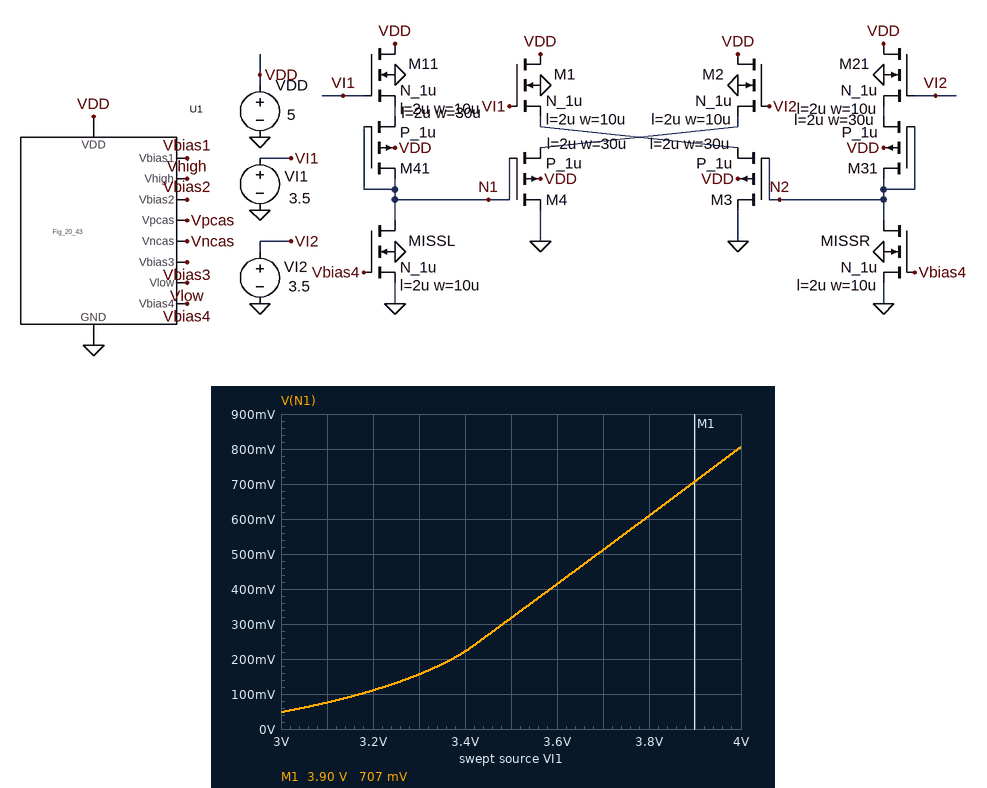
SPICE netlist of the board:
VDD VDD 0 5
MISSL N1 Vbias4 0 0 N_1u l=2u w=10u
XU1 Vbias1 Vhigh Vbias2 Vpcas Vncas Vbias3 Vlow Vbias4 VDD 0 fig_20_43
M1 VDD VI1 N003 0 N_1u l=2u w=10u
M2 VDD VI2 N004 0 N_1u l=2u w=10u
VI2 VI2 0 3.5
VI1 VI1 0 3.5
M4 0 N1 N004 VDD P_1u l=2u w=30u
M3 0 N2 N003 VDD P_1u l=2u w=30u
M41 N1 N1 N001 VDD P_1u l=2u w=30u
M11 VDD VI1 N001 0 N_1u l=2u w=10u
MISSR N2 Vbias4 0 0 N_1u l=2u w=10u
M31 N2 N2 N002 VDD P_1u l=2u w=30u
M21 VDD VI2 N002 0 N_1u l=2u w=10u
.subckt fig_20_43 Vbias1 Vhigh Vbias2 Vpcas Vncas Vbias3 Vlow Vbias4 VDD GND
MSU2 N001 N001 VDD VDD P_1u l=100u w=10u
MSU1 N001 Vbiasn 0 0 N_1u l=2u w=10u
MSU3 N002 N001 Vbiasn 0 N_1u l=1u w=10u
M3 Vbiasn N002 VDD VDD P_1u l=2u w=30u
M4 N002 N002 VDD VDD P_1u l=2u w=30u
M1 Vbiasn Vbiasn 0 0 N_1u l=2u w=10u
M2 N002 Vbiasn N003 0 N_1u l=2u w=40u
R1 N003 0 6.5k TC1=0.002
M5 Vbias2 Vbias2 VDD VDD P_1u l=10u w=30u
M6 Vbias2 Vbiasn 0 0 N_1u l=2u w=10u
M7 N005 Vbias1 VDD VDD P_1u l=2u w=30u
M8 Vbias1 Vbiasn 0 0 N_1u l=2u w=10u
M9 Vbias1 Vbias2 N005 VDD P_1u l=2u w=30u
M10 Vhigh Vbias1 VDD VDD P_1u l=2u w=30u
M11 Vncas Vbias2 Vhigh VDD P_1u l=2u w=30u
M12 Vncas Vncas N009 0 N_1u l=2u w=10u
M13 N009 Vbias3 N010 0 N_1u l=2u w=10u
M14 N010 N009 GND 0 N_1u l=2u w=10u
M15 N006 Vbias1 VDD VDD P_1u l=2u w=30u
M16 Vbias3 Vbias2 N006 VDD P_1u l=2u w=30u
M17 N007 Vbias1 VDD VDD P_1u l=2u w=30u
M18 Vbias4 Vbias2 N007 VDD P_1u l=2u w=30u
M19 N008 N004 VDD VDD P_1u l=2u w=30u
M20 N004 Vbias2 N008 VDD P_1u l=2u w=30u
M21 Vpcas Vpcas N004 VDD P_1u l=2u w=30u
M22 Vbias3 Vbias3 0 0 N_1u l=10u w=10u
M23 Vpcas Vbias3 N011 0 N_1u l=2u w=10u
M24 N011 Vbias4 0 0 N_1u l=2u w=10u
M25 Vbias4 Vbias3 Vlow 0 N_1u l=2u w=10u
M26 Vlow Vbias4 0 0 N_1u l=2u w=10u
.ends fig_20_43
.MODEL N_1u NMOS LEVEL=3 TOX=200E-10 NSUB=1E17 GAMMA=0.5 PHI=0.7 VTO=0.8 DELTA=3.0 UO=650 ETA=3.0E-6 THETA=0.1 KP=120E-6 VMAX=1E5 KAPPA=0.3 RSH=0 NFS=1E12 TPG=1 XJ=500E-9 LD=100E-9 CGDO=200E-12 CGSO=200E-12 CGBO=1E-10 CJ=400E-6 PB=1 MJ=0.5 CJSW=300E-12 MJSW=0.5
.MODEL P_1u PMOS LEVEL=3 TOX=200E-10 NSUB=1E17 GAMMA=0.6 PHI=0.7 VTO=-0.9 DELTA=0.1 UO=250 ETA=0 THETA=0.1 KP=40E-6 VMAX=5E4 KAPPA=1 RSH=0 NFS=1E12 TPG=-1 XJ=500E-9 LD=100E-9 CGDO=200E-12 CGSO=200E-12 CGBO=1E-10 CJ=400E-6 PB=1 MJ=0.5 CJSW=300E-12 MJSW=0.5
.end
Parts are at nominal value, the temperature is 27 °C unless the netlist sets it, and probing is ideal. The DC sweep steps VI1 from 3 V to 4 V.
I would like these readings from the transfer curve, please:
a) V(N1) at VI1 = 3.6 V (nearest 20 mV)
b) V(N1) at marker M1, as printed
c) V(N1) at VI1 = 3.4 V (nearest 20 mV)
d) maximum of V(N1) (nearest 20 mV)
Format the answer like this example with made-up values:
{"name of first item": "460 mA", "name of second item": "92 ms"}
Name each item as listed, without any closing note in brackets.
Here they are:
{"V(N1) at VI1 = 3.6 V": "420 mV", "V(N1) at marker M1, as printed": "707 mV", "V(N1) at VI1 = 3.4 V": "220 mV", "maximum of V(N1)": "800 mV"}
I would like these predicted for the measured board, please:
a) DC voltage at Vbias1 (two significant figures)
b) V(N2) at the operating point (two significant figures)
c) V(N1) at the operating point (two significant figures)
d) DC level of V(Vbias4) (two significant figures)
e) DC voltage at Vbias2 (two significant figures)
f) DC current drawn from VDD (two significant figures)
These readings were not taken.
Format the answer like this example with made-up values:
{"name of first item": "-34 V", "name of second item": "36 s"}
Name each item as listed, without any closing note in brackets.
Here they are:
{"DC voltage at Vbias1": "3.8 V", "V(N2) at the operating point": "320 mV", "V(N1) at the operating point": "320 mV", "DC level of V(Vbias4)": "1.1 V", "DC voltage at Vbias2": "3.4 V", "DC current drawn from VDD": "280 µA"}
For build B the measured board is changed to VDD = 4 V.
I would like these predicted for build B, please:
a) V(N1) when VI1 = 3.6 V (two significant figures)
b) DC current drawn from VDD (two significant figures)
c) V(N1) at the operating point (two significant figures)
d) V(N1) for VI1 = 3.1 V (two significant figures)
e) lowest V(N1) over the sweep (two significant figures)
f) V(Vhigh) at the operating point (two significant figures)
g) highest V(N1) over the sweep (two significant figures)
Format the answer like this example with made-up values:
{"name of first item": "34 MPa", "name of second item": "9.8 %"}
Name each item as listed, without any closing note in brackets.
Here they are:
{"V(N1) when VI1 = 3.6 V": "570 mV", "DC current drawn from VDD": "260 µA", "V(N1) at the operating point": "470 mV", "V(N1) for VI1 = 3.1 V": "130 mV", "lowest V(N1) over the sweep": "89 mV", "V(Vhigh) at the operating point": "3.7 V", "highest V(N1) over the sweep": "970 mV"}
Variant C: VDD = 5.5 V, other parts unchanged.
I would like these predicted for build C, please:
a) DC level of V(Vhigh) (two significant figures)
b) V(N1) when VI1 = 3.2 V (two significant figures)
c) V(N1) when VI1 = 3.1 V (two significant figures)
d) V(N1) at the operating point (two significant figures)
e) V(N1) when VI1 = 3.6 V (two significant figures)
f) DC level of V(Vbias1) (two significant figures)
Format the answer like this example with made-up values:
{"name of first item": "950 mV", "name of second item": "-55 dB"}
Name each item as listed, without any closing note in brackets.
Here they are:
{"DC level of V(Vhigh)": "5.2 V", "V(N1) when VI1 = 3.2 V": "87 mV", "V(N1) when VI1 = 3.1 V": "58 mV", "V(N1) at the operating point": "250 mV", "V(N1) when VI1 = 3.6 V": "350 mV", "DC level of V(Vbias1)": "4.3 V"}
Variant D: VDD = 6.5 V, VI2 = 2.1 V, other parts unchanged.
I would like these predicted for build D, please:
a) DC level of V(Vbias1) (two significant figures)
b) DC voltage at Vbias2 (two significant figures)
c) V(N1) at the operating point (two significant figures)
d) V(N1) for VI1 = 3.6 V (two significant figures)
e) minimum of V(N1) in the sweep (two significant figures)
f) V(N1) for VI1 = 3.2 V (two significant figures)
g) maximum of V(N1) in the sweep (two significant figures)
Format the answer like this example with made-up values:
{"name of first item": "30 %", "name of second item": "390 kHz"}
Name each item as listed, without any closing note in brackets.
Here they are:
{"DC level of V(Vbias1)": "5.3 V", "DC voltage at Vbias2": "4.9 V", "V(N1) at the operating point": "160 mV", "V(N1) for VI1 = 3.6 V": "230 mV", "minimum of V(N1) in the sweep": "15 mV", "V(N1) for VI1 = 3.2 V": "53 mV", "maximum of V(N1) in the sweep": "610 mV"}
